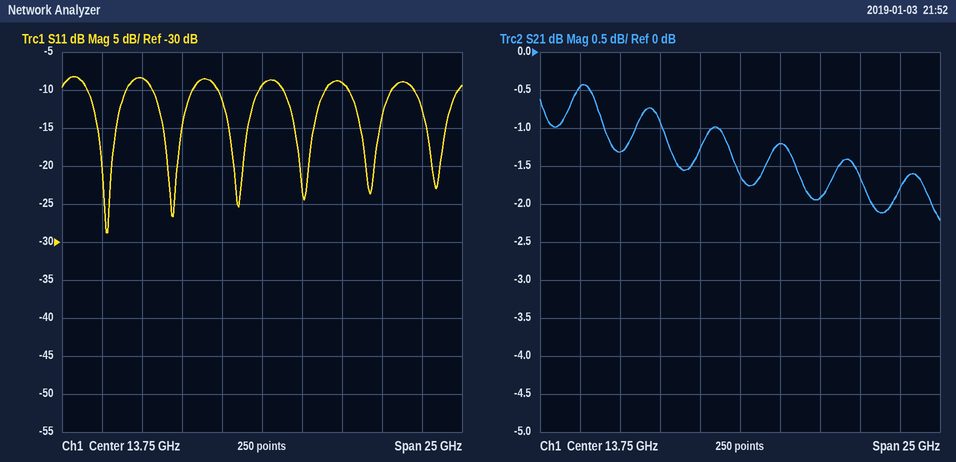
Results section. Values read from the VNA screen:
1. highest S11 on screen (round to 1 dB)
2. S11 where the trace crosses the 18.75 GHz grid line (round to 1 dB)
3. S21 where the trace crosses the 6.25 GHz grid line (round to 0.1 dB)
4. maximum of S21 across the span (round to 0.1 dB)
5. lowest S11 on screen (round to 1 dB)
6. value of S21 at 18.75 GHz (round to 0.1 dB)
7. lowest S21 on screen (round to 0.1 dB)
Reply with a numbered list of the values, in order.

1. -8 dB
2. -9 dB
3. -1.3 dB
4. -0.4 dB
5. -29 dB
6. -1.9 dB
7. -2.2 dB
